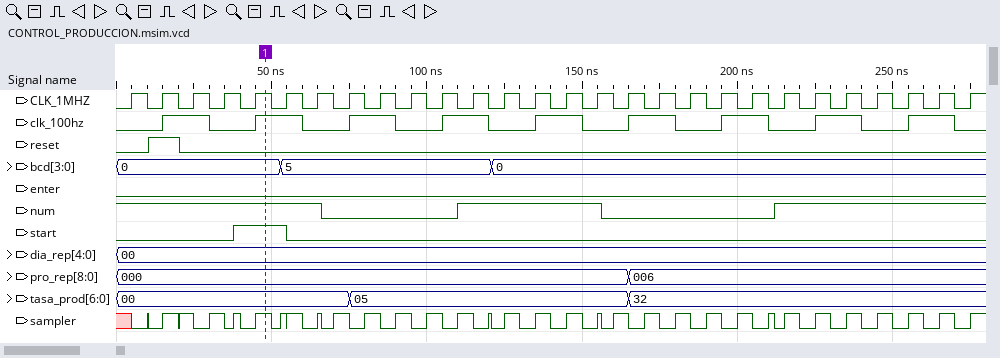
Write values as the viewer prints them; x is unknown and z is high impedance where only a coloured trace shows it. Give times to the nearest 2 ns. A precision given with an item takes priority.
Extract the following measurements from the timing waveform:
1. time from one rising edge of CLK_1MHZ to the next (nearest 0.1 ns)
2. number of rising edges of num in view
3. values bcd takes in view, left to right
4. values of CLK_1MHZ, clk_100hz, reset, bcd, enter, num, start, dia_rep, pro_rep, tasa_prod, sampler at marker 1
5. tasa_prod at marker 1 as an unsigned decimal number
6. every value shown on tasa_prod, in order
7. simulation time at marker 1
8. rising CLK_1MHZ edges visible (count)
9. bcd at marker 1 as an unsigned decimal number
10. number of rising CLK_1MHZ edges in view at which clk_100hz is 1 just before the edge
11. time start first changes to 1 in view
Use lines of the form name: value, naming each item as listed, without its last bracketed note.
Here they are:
time from one rising edge of CLK_1MHZ to the next: 10 ns
number of rising edges of num in view: 2
values bcd takes in view, left to right: 0, 5, 0
values of CLK_1MHZ, clk_100hz, reset, bcd, enter, num, start, dia_rep, pro_rep, tasa_prod, sampler at marker 1: CLK_1MHZ=1, clk_100hz=1, reset=0, bcd=0, enter=0, num=1, start=1, dia_rep=00, pro_rep=000, tasa_prod=00, sampler=1
tasa_prod at marker 1 as an unsigned decimal number: 0
every value shown on tasa_prod, in order: 00, 05, 32
simulation time at marker 1: 48 ns
rising CLK_1MHZ edges visible: 28
bcd at marker 1 as an unsigned decimal number: 0
number of rising CLK_1MHZ edges in view at which clk_100hz is 1 just before the edge: 9
time start first changes to 1 in view: 38 ns
